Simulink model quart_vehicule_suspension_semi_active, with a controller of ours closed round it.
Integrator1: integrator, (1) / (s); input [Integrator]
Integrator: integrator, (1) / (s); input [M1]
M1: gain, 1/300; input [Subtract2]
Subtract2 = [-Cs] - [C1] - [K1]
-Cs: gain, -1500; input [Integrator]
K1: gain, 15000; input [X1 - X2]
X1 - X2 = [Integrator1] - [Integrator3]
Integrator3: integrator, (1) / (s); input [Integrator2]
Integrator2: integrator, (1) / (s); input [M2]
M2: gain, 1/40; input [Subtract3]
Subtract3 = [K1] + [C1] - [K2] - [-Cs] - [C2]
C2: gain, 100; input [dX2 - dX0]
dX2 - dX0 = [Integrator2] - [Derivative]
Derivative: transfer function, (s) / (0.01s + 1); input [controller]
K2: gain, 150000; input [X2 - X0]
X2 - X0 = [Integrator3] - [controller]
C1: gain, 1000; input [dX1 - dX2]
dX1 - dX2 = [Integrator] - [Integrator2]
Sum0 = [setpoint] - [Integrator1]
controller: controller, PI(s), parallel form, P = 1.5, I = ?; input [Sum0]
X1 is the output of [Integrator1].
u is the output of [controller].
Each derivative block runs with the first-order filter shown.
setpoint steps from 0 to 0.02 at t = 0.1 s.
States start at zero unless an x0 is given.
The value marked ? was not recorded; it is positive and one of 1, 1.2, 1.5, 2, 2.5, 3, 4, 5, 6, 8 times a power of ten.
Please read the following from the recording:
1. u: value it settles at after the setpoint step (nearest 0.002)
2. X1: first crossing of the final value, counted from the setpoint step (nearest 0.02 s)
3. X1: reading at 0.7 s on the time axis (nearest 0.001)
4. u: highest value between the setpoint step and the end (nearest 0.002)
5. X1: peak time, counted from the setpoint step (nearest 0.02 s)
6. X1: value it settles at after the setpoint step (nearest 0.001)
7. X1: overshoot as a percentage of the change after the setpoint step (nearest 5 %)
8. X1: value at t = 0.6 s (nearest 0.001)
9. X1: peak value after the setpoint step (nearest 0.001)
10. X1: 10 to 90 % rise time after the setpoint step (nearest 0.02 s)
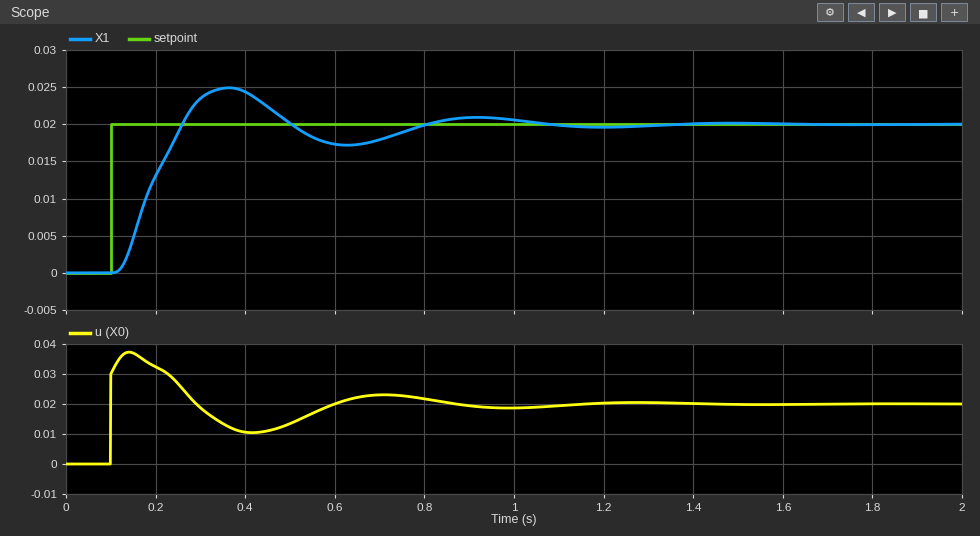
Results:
0.020
0.16 s
0.018
0.038
0.26 s
0.020
25 %
0.017
0.025
0.10 s
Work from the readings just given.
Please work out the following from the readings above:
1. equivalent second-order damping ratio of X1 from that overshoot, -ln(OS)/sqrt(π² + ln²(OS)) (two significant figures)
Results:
0.40
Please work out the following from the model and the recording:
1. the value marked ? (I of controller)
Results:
15
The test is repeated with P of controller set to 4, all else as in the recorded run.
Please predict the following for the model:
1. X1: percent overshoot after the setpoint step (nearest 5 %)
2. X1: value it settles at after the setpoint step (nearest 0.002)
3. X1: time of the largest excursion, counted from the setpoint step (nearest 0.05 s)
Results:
15 %
0.020
0.20 s
